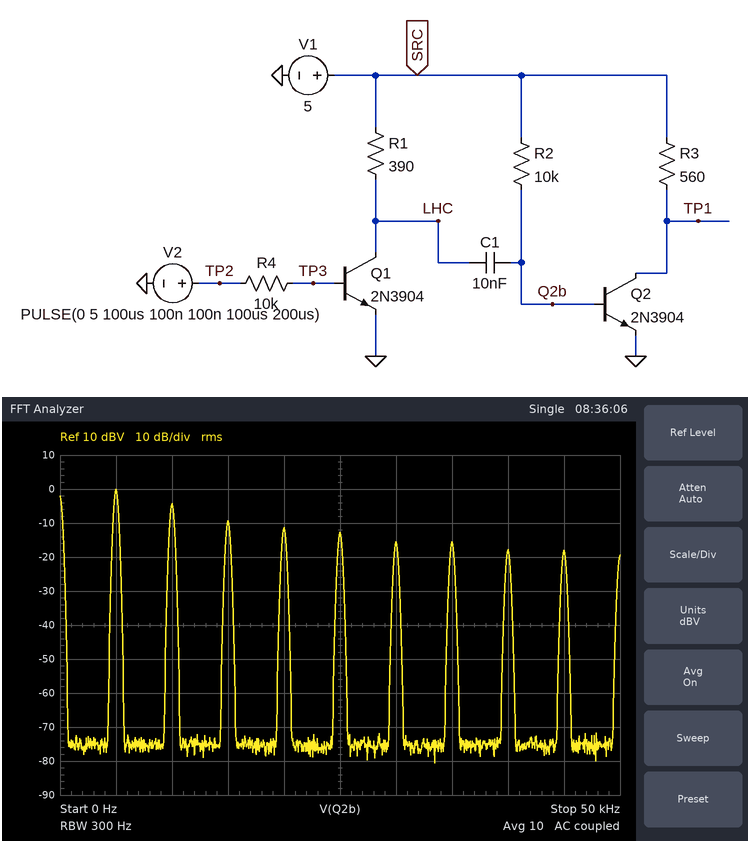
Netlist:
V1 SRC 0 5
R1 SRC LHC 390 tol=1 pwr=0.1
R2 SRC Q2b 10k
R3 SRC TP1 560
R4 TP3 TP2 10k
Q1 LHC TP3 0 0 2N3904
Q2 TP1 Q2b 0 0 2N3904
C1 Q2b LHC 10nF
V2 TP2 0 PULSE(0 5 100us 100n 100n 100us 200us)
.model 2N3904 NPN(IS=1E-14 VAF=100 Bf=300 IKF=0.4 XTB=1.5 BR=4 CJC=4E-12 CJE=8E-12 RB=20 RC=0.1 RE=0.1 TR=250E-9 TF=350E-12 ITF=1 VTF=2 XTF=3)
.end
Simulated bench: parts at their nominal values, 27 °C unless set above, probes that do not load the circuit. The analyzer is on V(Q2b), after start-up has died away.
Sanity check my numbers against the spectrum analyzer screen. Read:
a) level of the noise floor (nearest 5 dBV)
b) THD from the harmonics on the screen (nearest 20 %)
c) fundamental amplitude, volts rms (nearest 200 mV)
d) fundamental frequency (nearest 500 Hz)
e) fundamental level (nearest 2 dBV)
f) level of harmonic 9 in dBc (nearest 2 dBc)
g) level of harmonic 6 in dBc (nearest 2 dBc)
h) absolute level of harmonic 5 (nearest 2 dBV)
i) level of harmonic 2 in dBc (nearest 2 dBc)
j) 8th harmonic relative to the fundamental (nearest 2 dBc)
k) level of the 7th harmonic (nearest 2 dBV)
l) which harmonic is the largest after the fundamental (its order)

-75 dBV
80 %
1.0 V
5.0 kHz
0 dBV
-18 dBc
-16 dBc
-12 dBV
-4 dBc
-18 dBc
-16 dBV
2
